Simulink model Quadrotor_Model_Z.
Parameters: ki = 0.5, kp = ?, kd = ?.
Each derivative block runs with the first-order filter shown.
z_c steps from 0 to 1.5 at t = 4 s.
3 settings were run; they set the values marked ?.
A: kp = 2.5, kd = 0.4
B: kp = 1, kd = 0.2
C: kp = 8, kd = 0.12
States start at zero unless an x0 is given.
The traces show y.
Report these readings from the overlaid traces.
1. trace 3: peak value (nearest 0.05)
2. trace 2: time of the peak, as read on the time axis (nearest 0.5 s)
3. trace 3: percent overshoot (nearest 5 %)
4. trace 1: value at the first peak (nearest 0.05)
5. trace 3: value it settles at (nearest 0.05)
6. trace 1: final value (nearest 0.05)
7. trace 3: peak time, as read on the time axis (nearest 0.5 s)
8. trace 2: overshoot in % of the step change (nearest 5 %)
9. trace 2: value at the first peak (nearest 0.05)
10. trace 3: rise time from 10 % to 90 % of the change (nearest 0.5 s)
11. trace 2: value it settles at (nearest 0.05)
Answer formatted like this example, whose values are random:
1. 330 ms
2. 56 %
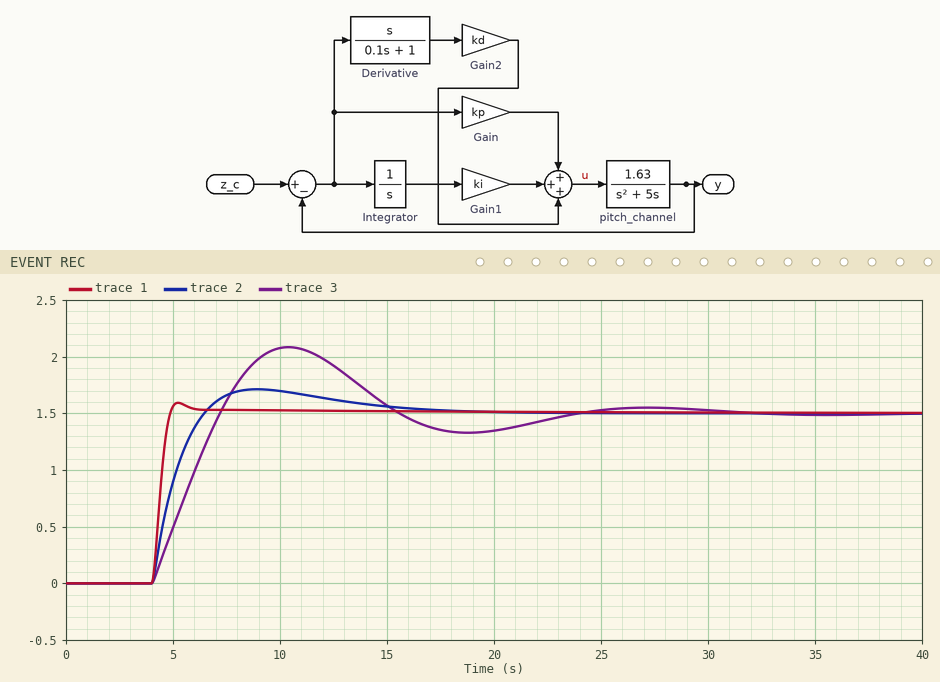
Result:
1. 2.10
2. 9.0 s
3. 40 %
4. 1.60
5. 1.50
6. 1.50
7. 10.5 s
8. 15 %
9. 1.70
10. 2.5 s
11. 1.50
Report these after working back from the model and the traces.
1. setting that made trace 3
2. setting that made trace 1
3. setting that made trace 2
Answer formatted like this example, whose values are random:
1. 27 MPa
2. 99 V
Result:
1. B
2. C
3. A
